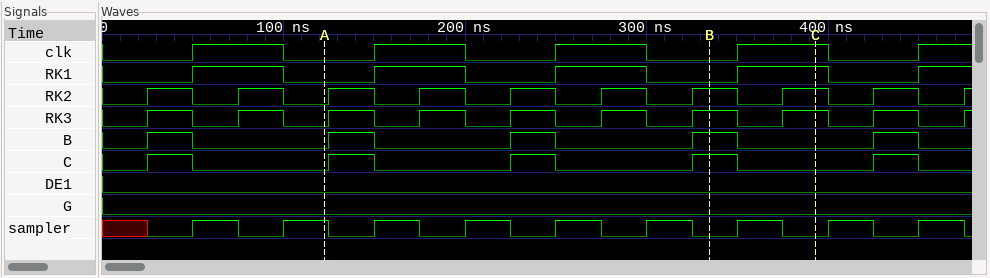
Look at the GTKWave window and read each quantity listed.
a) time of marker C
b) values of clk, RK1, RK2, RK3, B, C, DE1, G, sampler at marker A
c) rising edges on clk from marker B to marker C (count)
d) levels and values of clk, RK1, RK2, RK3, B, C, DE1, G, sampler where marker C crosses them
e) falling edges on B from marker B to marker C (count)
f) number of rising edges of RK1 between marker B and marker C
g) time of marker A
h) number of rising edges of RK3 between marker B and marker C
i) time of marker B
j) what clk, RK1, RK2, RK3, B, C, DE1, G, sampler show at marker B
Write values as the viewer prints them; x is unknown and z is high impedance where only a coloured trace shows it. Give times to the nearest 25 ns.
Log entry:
400 ns
clk=0, RK1=0, RK2=0, RK3=0, B=0, C=0, DE1=0, G=0, sampler=1
1
clk=1, RK1=1, RK2=1, RK3=1, B=0, C=0, DE1=0, G=0, sampler=0
1
1
125 ns
1
325 ns
clk=0, RK1=0, RK2=1, RK3=1, B=1, C=1, DE1=0, G=0, sampler=0
